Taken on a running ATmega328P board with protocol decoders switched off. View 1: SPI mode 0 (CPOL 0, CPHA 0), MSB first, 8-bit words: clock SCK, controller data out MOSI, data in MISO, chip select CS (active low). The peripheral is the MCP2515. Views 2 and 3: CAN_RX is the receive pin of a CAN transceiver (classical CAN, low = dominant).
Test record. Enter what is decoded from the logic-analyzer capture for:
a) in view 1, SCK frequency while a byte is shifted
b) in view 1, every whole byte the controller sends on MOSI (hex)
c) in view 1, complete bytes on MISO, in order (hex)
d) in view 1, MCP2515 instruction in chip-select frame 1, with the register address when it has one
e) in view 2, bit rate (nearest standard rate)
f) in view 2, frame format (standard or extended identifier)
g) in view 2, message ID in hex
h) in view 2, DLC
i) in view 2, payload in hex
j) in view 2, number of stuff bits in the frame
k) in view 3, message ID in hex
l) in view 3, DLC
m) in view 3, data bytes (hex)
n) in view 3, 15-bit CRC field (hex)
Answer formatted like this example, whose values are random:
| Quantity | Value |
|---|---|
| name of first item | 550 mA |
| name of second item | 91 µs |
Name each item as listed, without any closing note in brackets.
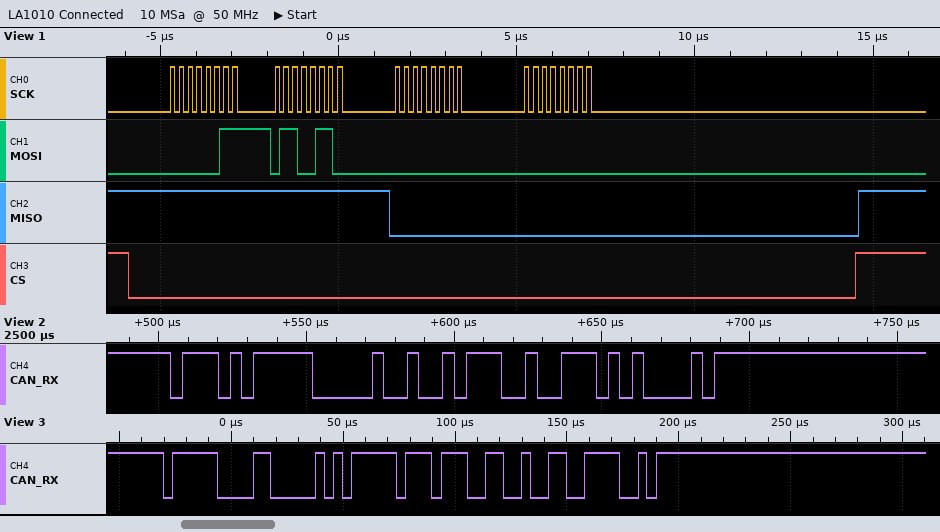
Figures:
| Quantity | Value |
|---|---|
| in view 1, SCK frequency while a byte is shifted | 4 MHz |
| in view 1, every whole byte the controller sends on MOSI | 03 66 00 00 |
| in view 1, complete bytes on MISO, in order | FF FF 00 00 |
| in view 1, MCP2515 instruction in chip-select frame 1, with the register address when it has one | READ 0x66 |
| in view 2, bit rate | 250 kbit/s |
| in view 2, frame format | standard |
| in view 2, message ID in hex | 0x75F |
| in view 2, DLC | 1 |
| in view 2, payload in hex | 2E |
| in view 2, number of stuff bits in the frame | 2 |
| in view 3, message ID in hex | 0x7C6 |
| in view 3, DLC | 2 |
| in view 3, data bytes | FF 73 |
| in view 3, 15-bit CRC field | 0x133C |
